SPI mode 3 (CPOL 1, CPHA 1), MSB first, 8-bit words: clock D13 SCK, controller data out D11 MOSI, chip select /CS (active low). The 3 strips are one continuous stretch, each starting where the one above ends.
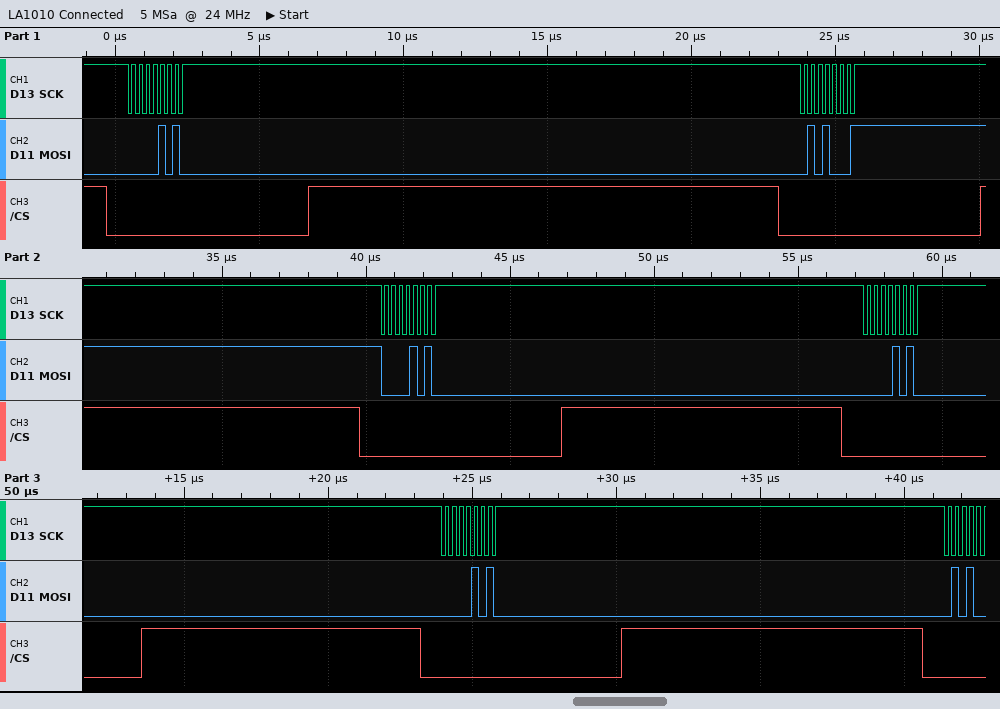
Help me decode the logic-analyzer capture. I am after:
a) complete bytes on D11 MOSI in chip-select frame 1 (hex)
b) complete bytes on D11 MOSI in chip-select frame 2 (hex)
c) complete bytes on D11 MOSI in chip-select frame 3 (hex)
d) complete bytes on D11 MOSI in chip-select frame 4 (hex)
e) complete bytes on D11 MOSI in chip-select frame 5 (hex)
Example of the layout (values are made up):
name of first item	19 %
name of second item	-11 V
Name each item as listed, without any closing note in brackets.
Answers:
complete bytes on D11 MOSI in chip-select frame 1	0A
complete bytes on D11 MOSI in chip-select frame 2	51
complete bytes on D11 MOSI in chip-select frame 3	0A
complete bytes on D11 MOSI in chip-select frame 4	0A
complete bytes on D11 MOSI in chip-select frame 5	0A
